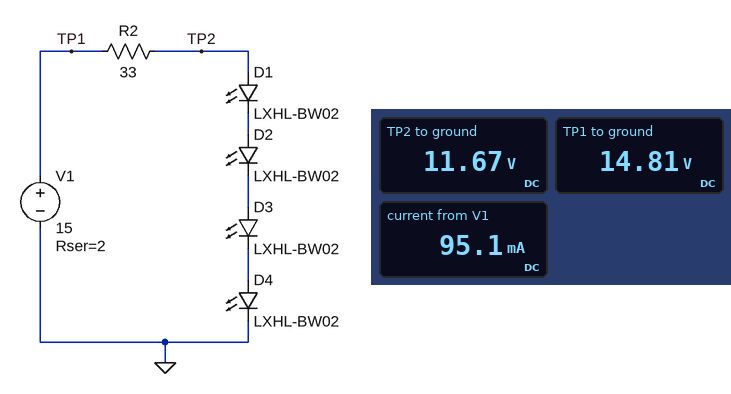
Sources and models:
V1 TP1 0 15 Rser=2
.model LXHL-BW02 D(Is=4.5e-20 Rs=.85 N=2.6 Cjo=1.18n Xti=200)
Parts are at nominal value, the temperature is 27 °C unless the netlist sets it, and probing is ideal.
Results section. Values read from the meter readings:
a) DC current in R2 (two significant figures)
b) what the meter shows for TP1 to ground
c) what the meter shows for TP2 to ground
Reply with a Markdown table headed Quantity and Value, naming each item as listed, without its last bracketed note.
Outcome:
| Quantity | Value |
|---|---|
| DC current in R2 | 95 mA |
| what the meter shows for TP1 to ground | 14.81 V |
| what the meter shows for TP2 to ground | 11.67 V |
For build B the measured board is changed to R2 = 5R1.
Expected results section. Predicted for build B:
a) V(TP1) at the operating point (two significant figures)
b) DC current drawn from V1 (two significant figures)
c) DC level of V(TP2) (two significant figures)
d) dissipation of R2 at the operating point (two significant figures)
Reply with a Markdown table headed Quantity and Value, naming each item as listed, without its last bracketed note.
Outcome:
| Quantity | Value |
|---|---|
| V(TP1) at the operating point | 14 V |
| DC current drawn from V1 | 320 mA |
| DC level of V(TP2) | 13 V |
| dissipation of R2 at the operating point | 510 mW |
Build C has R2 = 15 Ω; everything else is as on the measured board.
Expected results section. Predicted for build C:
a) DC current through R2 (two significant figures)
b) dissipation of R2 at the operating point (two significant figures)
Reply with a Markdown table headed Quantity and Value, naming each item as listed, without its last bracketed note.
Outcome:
| Quantity | Value |
|---|---|
| DC current through R2 | 170 mA |
| dissipation of R2 at the operating point | 440 mW |
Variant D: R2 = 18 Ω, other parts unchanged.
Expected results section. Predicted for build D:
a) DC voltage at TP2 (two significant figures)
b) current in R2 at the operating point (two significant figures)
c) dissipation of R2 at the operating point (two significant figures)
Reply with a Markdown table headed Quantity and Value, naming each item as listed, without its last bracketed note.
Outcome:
| Quantity | Value |
|---|---|
| DC voltage at TP2 | 12 V |
| current in R2 at the operating point | 150 mA |
| dissipation of R2 at the operating point | 410 mW |
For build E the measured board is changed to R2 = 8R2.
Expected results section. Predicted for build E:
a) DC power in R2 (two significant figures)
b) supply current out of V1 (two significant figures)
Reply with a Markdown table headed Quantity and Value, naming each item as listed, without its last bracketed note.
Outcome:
| Quantity | Value |
|---|---|
| DC power in R2 | 510 mW |
| supply current out of V1 | 250 mA |
